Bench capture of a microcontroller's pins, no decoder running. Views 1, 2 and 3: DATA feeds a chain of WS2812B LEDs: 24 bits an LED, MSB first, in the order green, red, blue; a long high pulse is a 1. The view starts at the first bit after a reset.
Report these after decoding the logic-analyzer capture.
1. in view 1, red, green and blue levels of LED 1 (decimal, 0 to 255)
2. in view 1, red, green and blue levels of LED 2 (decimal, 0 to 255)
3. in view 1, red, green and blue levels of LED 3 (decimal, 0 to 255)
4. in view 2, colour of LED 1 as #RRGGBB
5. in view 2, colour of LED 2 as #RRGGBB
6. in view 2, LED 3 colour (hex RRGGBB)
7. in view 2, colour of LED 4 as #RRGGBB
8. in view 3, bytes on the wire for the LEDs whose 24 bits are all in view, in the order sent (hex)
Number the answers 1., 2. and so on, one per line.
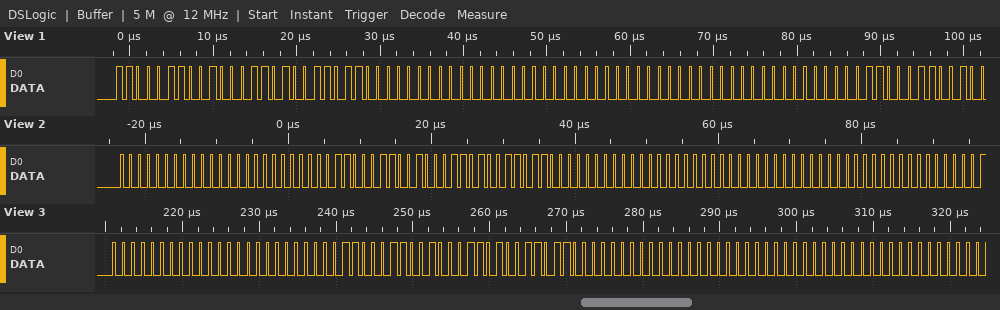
1. 70, 198, 155
2. 0, 0, 0
3. 0, 0, 0
4. #000000
5. #46C69B
6. #000000
7. #000000
8. 00 00 00 C6 46 9B 00 00 00
